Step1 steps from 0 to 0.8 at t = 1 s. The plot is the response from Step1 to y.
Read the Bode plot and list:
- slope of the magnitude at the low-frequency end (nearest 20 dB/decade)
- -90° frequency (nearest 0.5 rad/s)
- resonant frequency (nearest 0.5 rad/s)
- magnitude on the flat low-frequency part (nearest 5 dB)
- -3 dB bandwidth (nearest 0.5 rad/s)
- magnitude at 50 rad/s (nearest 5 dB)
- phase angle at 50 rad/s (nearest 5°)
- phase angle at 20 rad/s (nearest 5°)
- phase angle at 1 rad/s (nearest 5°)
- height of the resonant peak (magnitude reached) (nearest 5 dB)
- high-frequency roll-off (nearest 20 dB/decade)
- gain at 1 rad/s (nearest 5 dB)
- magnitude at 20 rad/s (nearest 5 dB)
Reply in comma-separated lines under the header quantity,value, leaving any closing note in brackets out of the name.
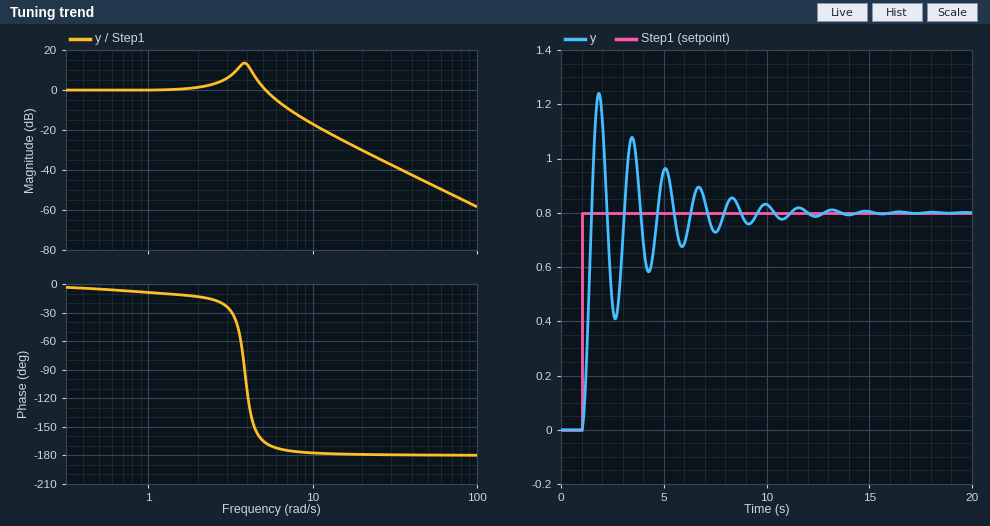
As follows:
quantity,value
slope of the magnitude at the low-frequency end,0 dB/decade
-90° frequency,4.0 rad/s
resonant frequency,4.0 rad/s
magnitude on the flat low-frequency part,0 dB
-3 dB bandwidth,5.5 rad/s
magnitude at 50 rad/s,-45 dB
phase angle at 50 rad/s,-180°
phase angle at 20 rad/s,-180°
phase angle at 1 rad/s,-10°
height of the resonant peak (magnitude reached),15 dB
high-frequency roll-off,-40 dB/decade
gain at 1 rad/s,0 dB
magnitude at 20 rad/s,-30 dB
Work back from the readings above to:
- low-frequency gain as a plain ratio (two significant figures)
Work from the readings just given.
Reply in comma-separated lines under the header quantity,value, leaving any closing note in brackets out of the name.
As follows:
quantity,value
low-frequency gain as a plain ratio,1.0
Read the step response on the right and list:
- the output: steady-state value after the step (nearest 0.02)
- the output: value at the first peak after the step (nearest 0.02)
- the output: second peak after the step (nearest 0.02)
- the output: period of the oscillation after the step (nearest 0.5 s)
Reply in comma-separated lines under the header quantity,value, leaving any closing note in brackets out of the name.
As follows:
quantity,value
the output: steady-state value after the step,0.80
the output: value at the first peak after the step,1.24
the output: second peak after the step,1.08
the output: period of the oscillation after the step,1.5 s
